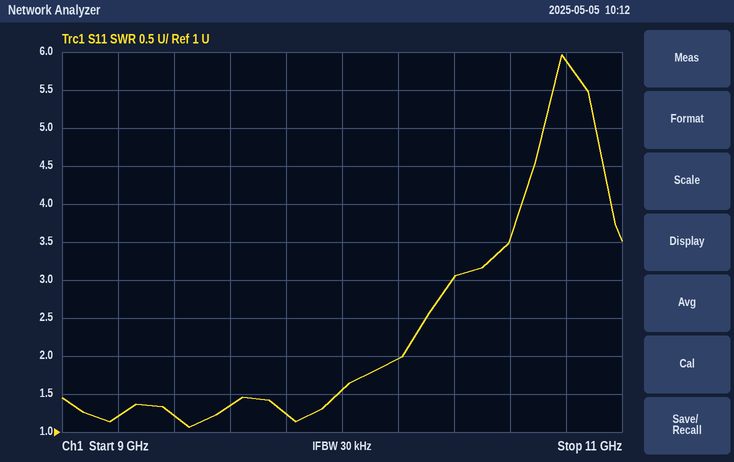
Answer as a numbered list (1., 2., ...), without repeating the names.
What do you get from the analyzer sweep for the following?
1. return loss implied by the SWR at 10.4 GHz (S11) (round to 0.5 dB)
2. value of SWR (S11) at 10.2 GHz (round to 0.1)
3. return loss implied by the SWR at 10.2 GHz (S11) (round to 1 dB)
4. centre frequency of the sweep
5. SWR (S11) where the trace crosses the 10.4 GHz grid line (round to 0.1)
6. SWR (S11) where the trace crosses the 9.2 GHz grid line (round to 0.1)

1. 6.0 dB
2. 2.0
3. 10 dB
4. 10 GHz
5. 3.0
6. 1.2
